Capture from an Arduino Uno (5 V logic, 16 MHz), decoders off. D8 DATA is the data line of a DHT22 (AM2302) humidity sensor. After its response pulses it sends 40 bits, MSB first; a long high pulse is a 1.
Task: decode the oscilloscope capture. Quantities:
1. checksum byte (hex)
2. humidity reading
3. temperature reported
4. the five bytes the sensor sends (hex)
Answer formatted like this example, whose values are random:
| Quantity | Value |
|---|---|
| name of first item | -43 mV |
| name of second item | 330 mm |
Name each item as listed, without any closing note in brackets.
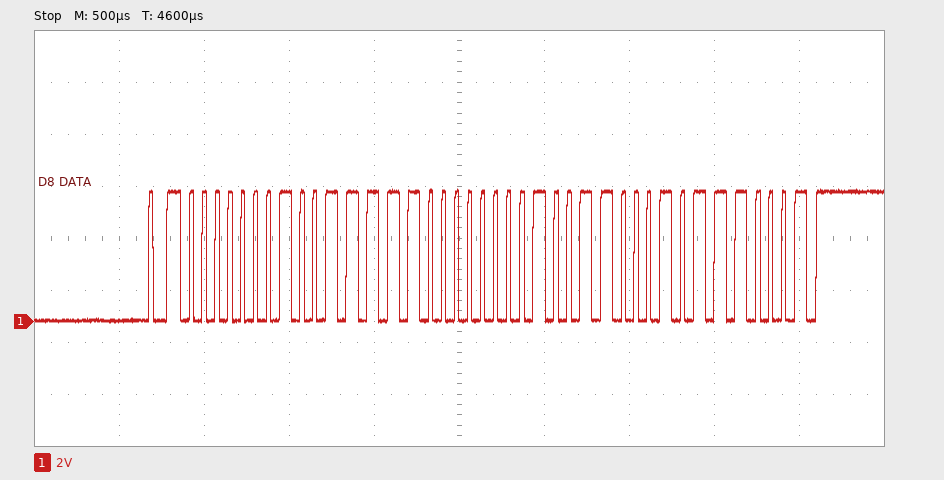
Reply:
| Quantity | Value |
|---|---|
| checksum byte | 0x71 |
| humidity reading | 31.8 % |
| temperature reported | 30.5 °C |
| the five bytes the sensor sends | 01 3E 01 31 71 |
